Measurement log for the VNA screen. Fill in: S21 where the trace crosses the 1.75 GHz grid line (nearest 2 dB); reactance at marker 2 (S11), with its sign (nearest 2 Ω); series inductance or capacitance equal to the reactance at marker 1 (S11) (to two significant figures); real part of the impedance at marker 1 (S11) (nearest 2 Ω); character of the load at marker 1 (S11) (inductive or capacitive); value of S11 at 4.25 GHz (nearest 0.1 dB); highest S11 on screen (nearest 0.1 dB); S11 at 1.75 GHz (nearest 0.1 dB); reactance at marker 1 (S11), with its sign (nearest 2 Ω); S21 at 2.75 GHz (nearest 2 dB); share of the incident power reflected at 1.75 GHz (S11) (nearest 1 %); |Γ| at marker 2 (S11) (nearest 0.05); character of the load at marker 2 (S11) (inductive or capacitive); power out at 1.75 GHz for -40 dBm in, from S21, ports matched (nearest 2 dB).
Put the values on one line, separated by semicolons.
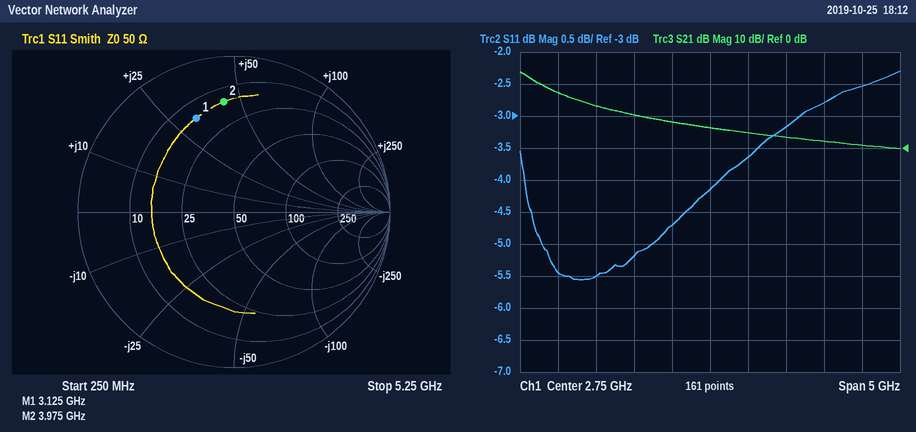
10 dB; +44 Ω; 1.6 nH; 16 Ω; inductive; -2.8 dB; -2.3 dB; -5.2 dB; +32 Ω; 6 dB; 30 %; 0.70; inductive; -30 dBm
